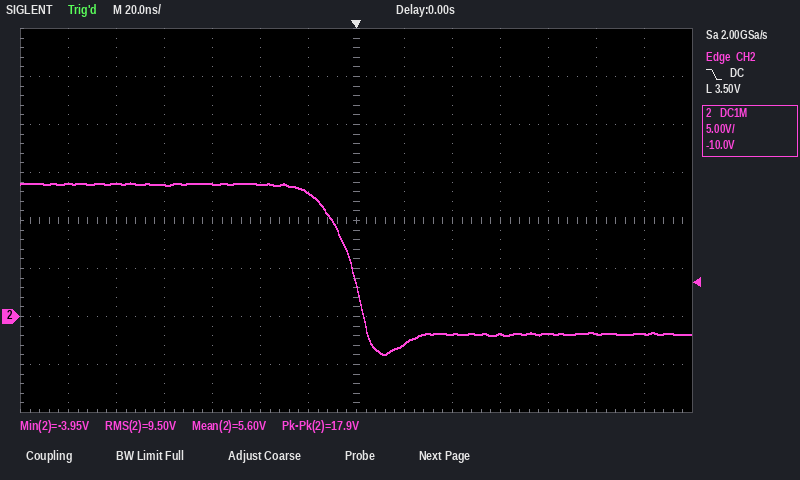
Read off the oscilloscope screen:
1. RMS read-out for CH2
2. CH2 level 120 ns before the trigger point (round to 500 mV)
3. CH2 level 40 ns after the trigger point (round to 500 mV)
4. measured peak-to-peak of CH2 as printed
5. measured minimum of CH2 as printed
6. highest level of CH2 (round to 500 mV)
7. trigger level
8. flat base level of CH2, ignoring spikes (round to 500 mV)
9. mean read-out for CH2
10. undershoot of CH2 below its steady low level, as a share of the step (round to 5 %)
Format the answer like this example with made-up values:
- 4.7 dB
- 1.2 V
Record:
- 9.50 V
- 14.0 V
- -2.0 V
- 17.9 V
- -3.95 V
- 14.0 V
- 3.50 V
- -2.0 V
- 5.60 V
- 15 %
